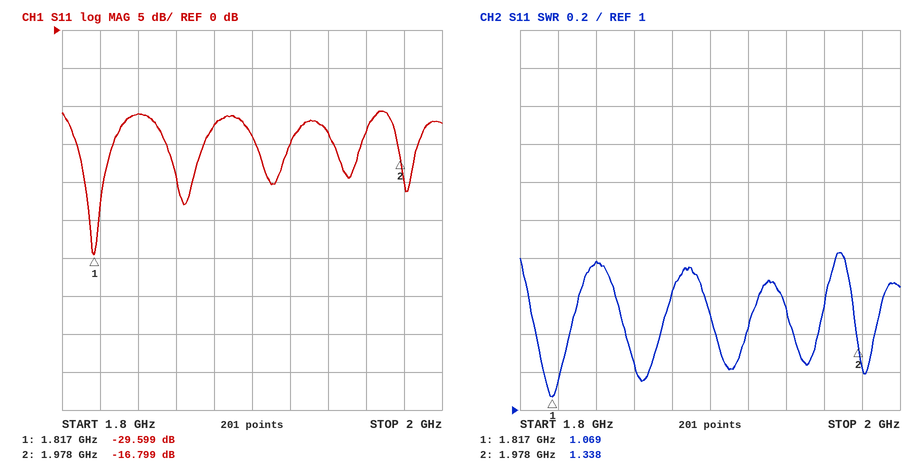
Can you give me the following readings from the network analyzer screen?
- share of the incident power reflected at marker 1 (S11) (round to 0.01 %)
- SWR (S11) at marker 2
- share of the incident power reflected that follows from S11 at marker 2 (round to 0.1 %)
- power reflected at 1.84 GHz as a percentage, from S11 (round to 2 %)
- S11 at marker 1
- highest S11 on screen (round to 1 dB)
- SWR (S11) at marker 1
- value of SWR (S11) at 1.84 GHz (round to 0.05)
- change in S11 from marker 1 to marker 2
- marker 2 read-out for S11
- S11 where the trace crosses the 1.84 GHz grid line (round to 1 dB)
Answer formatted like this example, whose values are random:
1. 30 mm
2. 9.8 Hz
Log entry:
1. 0.11 %
2. 1.338
3. 2.1 %
4. 8 %
5. -29.599 dB
6. -11 dB
7. 1.069
8. 1.80
9. 12.800 dB
10. -16.799 dB
11. -11 dB
